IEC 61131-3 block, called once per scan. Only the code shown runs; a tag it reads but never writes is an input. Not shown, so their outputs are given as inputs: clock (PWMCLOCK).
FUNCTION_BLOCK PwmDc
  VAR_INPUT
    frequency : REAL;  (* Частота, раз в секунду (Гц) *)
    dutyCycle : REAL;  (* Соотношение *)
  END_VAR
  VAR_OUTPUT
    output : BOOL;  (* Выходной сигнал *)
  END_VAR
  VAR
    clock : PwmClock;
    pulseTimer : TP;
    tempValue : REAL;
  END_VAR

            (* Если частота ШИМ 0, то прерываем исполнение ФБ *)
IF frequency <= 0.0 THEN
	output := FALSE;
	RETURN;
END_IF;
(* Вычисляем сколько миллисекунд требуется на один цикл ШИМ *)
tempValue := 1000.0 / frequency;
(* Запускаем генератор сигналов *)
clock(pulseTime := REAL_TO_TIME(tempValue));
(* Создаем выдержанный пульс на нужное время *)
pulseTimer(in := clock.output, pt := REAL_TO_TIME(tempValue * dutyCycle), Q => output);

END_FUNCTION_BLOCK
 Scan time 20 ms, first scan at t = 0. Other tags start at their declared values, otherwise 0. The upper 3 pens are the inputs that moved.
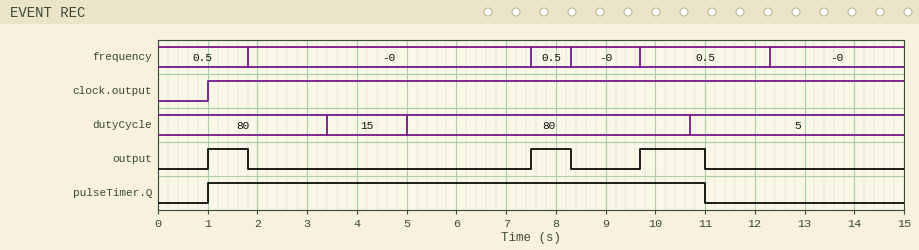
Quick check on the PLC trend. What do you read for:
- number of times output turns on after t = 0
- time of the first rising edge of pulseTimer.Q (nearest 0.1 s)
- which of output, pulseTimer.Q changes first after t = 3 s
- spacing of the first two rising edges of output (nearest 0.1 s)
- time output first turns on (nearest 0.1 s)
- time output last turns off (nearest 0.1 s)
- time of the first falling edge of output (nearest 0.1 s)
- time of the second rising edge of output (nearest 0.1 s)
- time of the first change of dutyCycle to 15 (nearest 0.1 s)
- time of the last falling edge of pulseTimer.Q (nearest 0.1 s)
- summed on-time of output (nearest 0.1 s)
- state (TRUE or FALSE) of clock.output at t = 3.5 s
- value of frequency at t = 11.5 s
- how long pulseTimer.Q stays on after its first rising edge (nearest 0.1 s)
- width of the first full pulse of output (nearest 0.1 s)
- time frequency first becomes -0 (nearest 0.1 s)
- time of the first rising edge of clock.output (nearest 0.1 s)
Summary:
3
1.0 s
output
6.5 s
1.0 s
11.0 s
1.8 s
7.5 s
3.4 s
11.0 s
2.9 s
TRUE
0.5
10.0 s
0.8 s
1.8 s
1.0 s
